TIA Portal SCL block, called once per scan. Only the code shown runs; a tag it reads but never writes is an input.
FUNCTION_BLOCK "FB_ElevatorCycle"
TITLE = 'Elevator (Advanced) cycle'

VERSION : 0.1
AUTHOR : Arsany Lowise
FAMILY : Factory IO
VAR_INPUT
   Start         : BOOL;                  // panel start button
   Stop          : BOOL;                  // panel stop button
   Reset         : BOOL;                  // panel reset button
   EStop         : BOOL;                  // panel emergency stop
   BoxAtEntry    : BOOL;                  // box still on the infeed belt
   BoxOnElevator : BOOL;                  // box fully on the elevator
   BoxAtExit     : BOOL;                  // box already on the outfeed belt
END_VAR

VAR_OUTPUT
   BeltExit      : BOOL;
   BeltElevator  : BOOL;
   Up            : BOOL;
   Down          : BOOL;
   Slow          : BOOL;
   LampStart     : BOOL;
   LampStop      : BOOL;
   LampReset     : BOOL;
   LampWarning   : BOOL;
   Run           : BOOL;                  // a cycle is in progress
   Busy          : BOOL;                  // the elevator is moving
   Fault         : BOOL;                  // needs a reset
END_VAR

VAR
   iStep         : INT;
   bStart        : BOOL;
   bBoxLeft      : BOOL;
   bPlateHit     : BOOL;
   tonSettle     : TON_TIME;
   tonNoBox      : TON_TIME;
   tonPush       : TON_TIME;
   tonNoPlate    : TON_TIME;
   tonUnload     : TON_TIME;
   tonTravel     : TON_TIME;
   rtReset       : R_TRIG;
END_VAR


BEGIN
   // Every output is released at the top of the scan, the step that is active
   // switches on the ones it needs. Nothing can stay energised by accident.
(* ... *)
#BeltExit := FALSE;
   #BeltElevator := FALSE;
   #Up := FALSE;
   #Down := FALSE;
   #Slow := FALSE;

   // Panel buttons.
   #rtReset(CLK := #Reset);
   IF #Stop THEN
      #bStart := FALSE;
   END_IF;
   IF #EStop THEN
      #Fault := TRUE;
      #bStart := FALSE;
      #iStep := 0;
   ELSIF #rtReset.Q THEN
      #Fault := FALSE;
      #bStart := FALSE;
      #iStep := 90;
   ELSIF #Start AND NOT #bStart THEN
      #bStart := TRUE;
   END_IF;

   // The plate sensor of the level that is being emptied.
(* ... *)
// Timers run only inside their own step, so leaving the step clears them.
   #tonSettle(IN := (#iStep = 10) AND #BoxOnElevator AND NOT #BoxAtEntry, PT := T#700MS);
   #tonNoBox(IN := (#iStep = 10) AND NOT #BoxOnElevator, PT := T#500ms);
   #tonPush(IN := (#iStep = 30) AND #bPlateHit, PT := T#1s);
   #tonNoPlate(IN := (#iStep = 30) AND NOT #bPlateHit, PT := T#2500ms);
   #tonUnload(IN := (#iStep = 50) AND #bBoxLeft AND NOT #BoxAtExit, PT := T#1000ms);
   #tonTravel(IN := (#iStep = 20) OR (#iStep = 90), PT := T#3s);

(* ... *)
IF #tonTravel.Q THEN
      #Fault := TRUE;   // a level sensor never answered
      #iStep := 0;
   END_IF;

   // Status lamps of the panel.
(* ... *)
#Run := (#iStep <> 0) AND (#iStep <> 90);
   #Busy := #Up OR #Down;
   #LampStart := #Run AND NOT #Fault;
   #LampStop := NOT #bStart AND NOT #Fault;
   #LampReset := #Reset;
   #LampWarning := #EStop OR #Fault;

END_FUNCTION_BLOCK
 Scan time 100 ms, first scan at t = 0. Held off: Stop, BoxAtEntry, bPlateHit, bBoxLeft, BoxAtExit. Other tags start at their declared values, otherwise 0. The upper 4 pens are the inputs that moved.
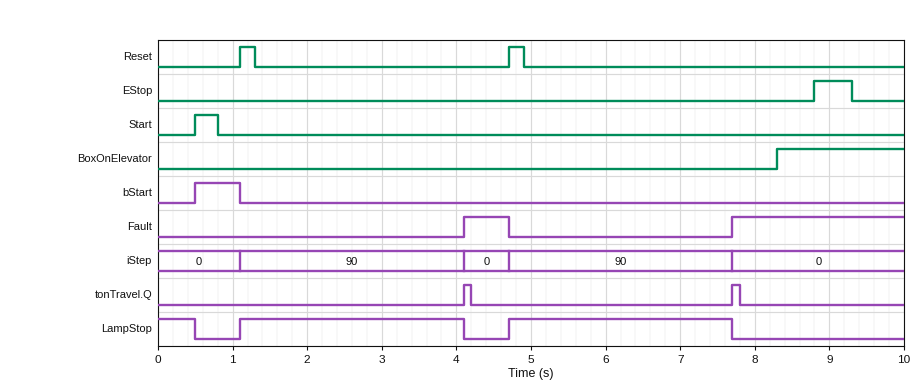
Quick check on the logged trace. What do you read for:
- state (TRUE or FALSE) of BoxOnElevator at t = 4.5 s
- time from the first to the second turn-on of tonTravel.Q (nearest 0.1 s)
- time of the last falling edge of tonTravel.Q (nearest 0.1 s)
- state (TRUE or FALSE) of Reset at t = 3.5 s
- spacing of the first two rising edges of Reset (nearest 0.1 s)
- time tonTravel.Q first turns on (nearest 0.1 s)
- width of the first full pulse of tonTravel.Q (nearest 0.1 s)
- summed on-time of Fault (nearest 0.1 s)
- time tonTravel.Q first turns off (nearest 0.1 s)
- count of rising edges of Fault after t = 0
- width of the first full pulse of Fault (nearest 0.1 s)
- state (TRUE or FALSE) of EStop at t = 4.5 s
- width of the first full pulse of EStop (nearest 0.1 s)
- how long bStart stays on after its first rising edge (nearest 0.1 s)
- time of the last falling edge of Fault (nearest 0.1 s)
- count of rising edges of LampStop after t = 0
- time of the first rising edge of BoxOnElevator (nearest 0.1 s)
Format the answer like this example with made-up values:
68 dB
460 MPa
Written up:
FALSE
3.6 s
7.8 s
FALSE
3.6 s
4.1 s
0.1 s
2.9 s
4.2 s
2
0.6 s
FALSE
0.5 s
0.6 s
4.7 s
2
8.3 s
